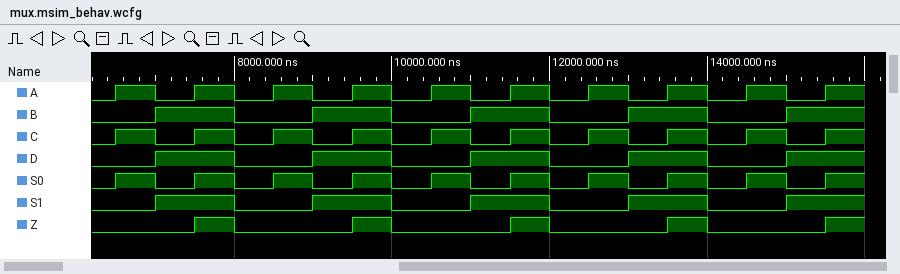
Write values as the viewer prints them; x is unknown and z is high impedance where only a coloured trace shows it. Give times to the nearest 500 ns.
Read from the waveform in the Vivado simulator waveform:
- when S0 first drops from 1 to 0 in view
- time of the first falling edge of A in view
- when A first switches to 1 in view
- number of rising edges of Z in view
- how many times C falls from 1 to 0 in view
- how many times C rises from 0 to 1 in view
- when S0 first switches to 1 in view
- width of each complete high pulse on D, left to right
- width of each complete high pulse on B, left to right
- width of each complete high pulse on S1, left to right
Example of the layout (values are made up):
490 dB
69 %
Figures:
7000 ns
7000 ns
6500 ns
5
9
10
6500 ns
1000 ns, 1000 ns, 1000 ns, 1000 ns
1000 ns, 1000 ns, 1000 ns, 1000 ns
1000 ns, 1000 ns, 1000 ns, 1000 ns
